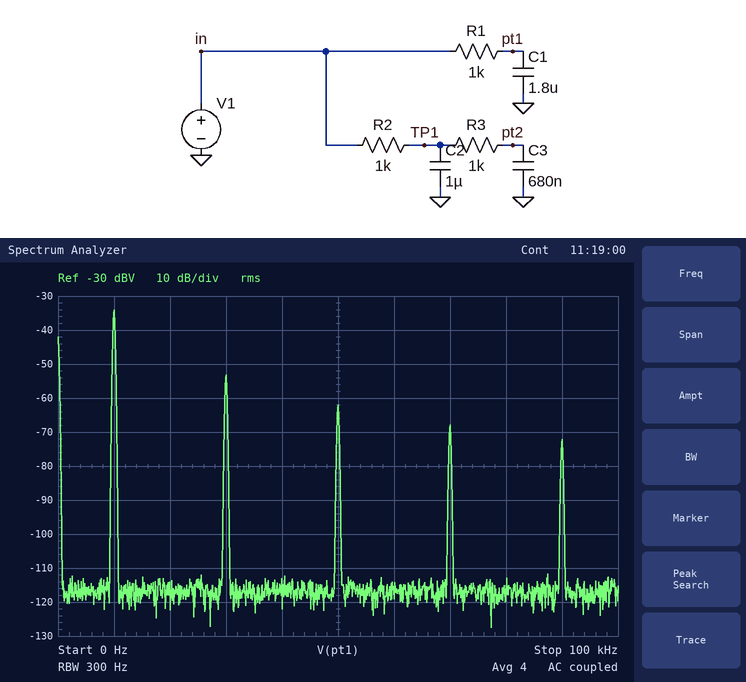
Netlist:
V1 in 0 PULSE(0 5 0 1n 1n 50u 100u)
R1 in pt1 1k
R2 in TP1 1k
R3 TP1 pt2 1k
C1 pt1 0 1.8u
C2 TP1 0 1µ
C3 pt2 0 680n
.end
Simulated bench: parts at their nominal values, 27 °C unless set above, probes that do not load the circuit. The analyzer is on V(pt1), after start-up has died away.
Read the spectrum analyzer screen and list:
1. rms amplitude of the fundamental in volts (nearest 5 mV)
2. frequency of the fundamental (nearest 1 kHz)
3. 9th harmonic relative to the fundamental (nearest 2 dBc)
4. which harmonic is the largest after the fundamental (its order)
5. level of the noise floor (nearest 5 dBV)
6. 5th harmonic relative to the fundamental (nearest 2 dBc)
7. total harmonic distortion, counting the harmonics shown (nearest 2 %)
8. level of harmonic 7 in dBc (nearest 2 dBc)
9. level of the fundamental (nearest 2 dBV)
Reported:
20 mV
10 kHz
-38 dBc
3
-115 dBV
-28 dBc
12 %
-34 dBc
-34 dBV
